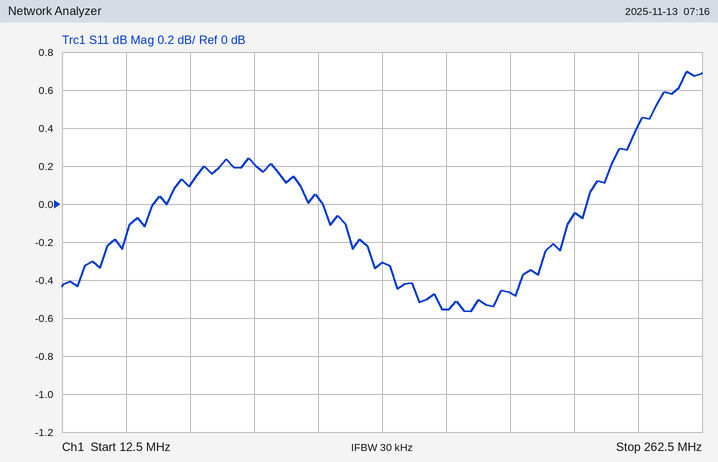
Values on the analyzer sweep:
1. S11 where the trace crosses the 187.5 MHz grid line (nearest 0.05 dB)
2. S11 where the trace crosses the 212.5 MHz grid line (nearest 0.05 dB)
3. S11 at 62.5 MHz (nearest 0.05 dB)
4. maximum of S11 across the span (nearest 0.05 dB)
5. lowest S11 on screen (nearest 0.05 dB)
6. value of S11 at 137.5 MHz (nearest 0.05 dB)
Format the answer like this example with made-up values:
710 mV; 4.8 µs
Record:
-0.45 dB; -0.05 dB; 0.10 dB; 0.70 dB; -0.55 dB; -0.30 dB
